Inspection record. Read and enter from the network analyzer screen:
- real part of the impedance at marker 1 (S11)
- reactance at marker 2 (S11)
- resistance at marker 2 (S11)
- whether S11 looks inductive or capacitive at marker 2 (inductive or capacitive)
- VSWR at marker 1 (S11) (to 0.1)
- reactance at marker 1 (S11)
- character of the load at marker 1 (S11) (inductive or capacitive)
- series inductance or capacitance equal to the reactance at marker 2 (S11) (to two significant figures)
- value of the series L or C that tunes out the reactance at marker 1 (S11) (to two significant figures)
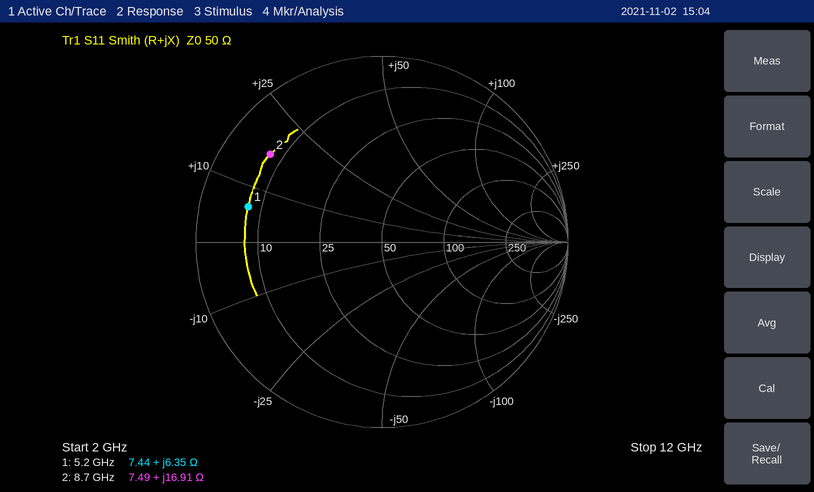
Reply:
7.44 Ω
+16.91 Ω
7.49 Ω
inductive
6.8
+6.35 Ω
inductive
310 pH
4.8 pF
